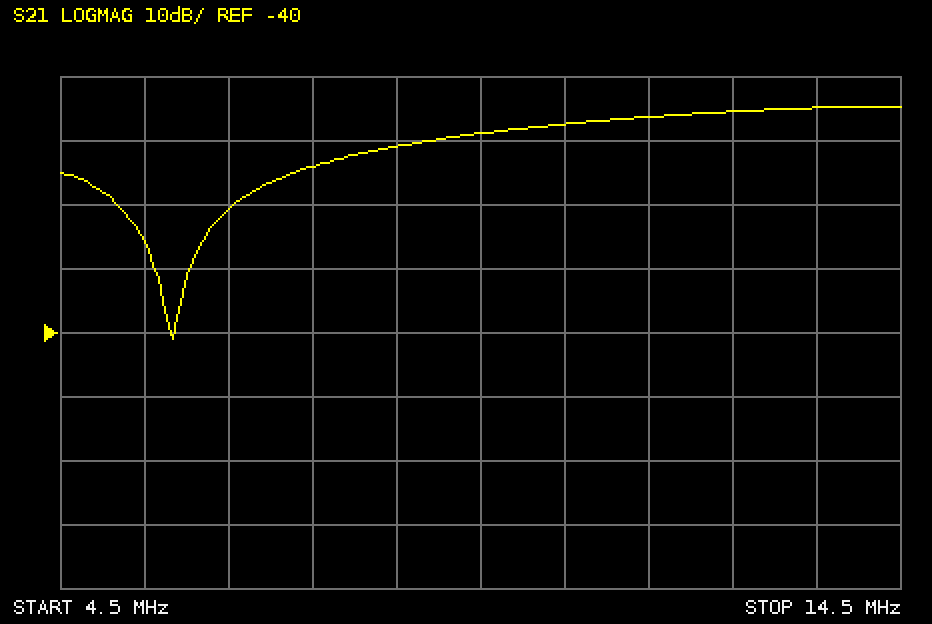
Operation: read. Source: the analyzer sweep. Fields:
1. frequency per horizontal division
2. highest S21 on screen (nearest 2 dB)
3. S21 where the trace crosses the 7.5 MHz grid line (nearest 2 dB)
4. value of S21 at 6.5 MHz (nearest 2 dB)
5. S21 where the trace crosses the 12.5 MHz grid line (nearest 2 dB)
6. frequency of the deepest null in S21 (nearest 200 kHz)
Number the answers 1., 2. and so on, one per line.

1. 1 MHz
2. -4 dB
3. -14 dB
4. -20 dB
5. -6 dB
6. 5.8 MHz
